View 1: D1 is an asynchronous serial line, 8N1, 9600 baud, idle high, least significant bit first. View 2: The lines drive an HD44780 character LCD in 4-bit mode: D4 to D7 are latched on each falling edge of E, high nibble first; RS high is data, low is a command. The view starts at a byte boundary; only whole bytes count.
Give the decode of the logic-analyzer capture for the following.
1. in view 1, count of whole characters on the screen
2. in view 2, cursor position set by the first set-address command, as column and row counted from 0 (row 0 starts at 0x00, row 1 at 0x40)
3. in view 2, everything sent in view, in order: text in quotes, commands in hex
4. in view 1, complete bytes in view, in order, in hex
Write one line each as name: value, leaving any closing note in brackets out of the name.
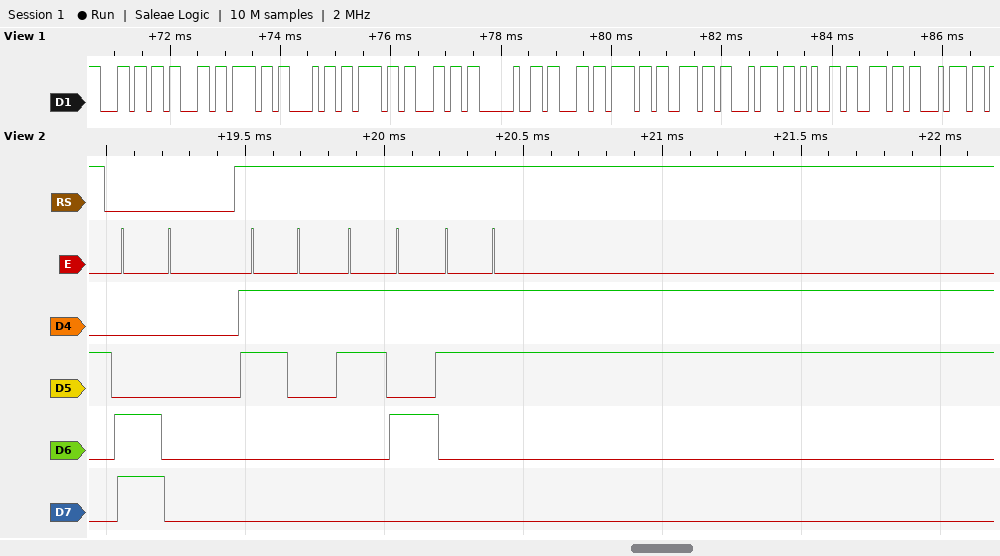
in view 1, count of whole characters on the screen: 14
in view 2, cursor position set by the first set-address command, as column and row counted from 0: column 0, row 1
in view 2, everything sent in view, in order: text in quotes, commands in hex: 0xC0 "153"
in view 1, complete bytes in view, in order, in hex: 6C 63 6F 68 6F 6C 20 63 6F 6E 74 65 6E 74
